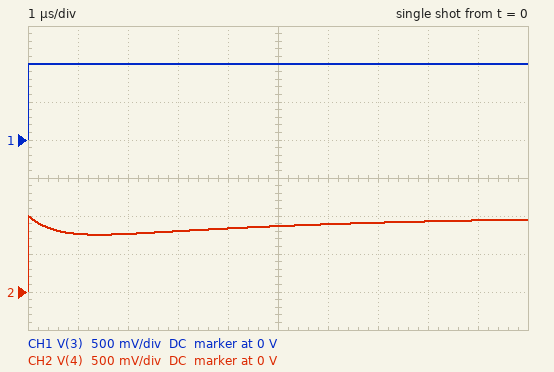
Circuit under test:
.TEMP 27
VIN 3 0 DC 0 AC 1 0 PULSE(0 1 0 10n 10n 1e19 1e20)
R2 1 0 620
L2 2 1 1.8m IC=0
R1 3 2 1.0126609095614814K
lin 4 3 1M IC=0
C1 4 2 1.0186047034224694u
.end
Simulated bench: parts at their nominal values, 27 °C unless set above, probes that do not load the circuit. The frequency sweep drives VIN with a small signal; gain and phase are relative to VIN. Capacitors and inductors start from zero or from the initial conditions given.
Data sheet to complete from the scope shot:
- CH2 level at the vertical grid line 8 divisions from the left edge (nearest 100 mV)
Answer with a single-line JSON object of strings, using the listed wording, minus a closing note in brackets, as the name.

{"CH2 level at the vertical grid line 8 divisions from the left edge": "900 mV"}
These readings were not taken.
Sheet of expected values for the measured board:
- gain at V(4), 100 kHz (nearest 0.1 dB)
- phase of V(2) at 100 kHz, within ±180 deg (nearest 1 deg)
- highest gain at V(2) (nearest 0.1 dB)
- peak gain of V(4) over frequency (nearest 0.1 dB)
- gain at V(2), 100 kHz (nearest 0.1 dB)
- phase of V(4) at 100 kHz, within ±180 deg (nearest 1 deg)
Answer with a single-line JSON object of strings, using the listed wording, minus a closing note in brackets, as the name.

{"gain at V(4), 100 kHz": "-3.0 dB", "phase of V(2) at 100 kHz, within ±180 deg": "1 deg", "highest gain at V(2)": "0 dB", "peak gain of V(4) over frequency": "0 dB", "gain at V(2), 100 kHz": "-3.0 dB", "phase of V(4) at 100 kHz, within ±180 deg": "1 deg"}
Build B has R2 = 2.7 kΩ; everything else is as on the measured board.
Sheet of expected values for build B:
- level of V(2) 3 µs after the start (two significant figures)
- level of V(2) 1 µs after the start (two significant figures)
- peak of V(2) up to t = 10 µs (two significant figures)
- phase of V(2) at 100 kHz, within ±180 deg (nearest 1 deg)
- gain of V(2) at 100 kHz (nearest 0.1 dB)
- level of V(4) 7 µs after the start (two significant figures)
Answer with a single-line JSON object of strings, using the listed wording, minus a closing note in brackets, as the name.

{"level of V(2) 3 µs after the start": "950 mV", "level of V(2) 1 µs after the start": "860 mV", "peak of V(2) up to t = 10 µs": "1.0 V", "phase of V(2) at 100 kHz, within ±180 deg": "-5 deg", "gain of V(2) at 100 kHz": "-1.2 dB", "level of V(4) 7 µs after the start": "1.0 V"}
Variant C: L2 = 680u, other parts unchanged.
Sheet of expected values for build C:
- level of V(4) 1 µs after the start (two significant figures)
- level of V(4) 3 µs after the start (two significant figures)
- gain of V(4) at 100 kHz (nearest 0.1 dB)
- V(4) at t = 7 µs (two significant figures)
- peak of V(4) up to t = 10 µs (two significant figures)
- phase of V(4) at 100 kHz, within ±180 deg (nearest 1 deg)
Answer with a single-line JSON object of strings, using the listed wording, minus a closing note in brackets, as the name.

{"level of V(4) 1 µs after the start": "630 mV", "level of V(4) 3 µs after the start": "780 mV", "gain of V(4) at 100 kHz": "-4.5 dB", "V(4) at t = 7 µs": "940 mV", "peak of V(4) up to t = 10 µs": "990 mV", "phase of V(4) at 100 kHz, within ±180 deg": "-10 deg"}
